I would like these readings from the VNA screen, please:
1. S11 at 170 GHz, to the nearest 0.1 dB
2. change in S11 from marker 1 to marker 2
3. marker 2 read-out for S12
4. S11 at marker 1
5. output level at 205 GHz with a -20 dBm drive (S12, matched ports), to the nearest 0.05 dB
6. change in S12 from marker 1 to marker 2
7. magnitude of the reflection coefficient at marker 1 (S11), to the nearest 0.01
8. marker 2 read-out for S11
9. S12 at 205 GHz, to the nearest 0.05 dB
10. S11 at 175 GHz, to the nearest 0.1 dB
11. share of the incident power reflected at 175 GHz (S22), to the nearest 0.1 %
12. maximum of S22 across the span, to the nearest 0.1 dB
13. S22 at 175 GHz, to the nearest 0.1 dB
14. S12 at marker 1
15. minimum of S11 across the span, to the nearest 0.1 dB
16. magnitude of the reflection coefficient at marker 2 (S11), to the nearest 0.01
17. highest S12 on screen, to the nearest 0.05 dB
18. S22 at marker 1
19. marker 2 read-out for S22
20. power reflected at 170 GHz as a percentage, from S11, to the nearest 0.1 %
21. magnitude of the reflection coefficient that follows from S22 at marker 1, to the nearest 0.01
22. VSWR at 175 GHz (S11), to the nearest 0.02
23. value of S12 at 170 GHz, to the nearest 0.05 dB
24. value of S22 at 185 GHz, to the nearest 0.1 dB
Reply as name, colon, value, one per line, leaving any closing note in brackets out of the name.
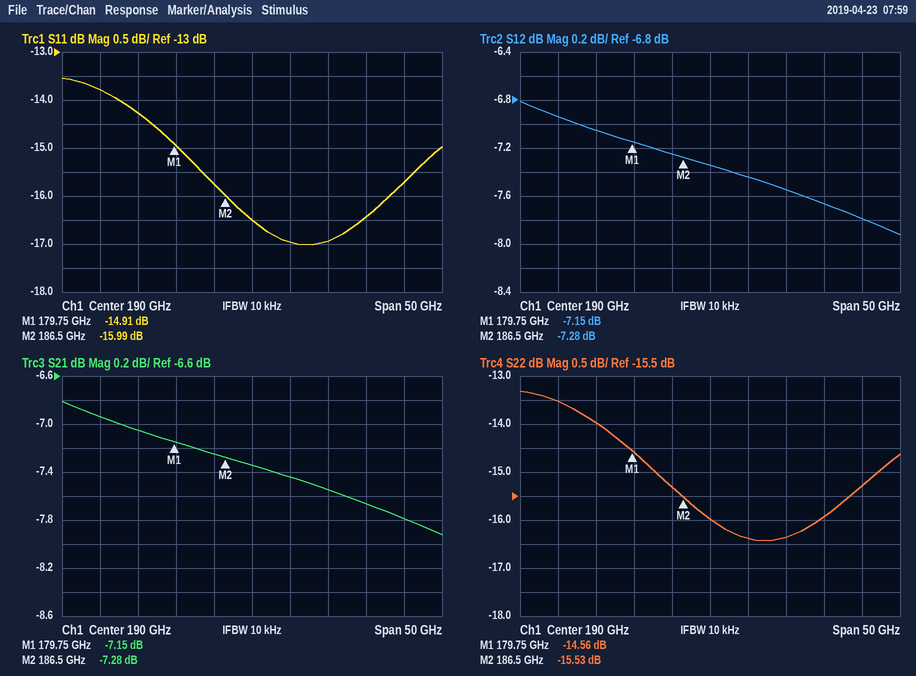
S11 at 170 GHz, to the nearest 0.1 dB: -13.8 dB
change in S11 from marker 1 to marker 2: -1.08 dB
marker 2 read-out for S12: -7.28 dB
S11 at marker 1: -14.91 dB
output level at 205 GHz with a -20 dBm drive (S12, matched ports), to the nearest 0.05 dB: -27.65 dBm
change in S12 from marker 1 to marker 2: -0.13 dB
magnitude of the reflection coefficient at marker 1 (S11), to the nearest 0.01: 0.18
marker 2 read-out for S11: -15.99 dB
S12 at 205 GHz, to the nearest 0.05 dB: -7.65 dB
S11 at 175 GHz, to the nearest 0.1 dB: -14.3 dB
share of the incident power reflected at 175 GHz (S22), to the nearest 0.1 %: 4.0 %
maximum of S22 across the span, to the nearest 0.1 dB: -13.3 dB
S22 at 175 GHz, to the nearest 0.1 dB: -14.0 dB
S12 at marker 1: -7.15 dB
minimum of S11 across the span, to the nearest 0.1 dB: -17.0 dB
magnitude of the reflection coefficient at marker 2 (S11), to the nearest 0.01: 0.16
highest S12 on screen, to the nearest 0.05 dB: -6.80 dB
S22 at marker 1: -14.56 dB
marker 2 read-out for S22: -15.53 dB
power reflected at 170 GHz as a percentage, from S11, to the nearest 0.1 %: 4.2 %
magnitude of the reflection coefficient that follows from S22 at marker 1, to the nearest 0.01: 0.19
VSWR at 175 GHz (S11), to the nearest 0.02: 1.48
value of S12 at 170 GHz, to the nearest 0.05 dB: -6.95 dB
value of S22 at 185 GHz, to the nearest 0.1 dB: -15.3 dB
